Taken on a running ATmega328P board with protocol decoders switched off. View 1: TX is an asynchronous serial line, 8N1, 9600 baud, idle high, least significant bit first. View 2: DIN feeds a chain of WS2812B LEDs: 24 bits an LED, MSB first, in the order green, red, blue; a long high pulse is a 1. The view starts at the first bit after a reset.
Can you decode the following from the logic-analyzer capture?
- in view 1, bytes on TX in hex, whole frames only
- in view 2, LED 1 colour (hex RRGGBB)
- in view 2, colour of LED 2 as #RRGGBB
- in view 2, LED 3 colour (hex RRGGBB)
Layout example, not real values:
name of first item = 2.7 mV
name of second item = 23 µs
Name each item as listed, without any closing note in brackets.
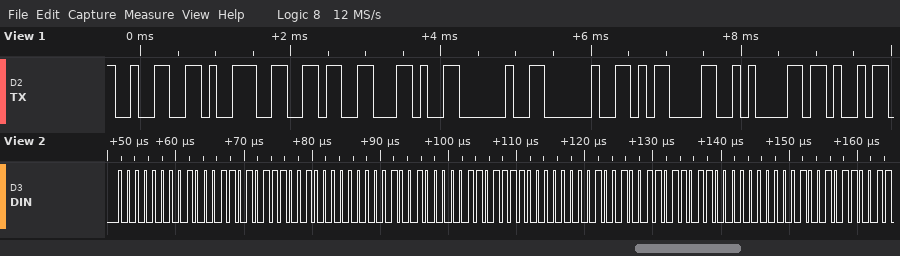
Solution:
in view 1, bytes on TX in hex, whole frames only = 32 39 36 2C 20 20 0D 0A 4B
in view 2, LED 1 colour = #8D0072
in view 2, colour of LED 2 as #RRGGBB = #90006F
in view 2, LED 3 colour = #93006C
